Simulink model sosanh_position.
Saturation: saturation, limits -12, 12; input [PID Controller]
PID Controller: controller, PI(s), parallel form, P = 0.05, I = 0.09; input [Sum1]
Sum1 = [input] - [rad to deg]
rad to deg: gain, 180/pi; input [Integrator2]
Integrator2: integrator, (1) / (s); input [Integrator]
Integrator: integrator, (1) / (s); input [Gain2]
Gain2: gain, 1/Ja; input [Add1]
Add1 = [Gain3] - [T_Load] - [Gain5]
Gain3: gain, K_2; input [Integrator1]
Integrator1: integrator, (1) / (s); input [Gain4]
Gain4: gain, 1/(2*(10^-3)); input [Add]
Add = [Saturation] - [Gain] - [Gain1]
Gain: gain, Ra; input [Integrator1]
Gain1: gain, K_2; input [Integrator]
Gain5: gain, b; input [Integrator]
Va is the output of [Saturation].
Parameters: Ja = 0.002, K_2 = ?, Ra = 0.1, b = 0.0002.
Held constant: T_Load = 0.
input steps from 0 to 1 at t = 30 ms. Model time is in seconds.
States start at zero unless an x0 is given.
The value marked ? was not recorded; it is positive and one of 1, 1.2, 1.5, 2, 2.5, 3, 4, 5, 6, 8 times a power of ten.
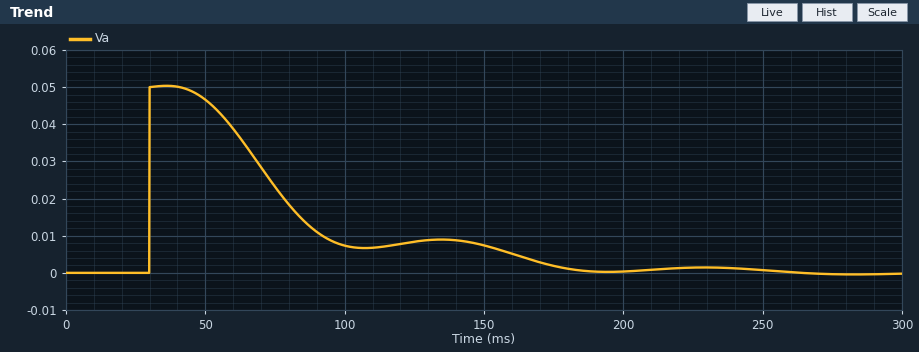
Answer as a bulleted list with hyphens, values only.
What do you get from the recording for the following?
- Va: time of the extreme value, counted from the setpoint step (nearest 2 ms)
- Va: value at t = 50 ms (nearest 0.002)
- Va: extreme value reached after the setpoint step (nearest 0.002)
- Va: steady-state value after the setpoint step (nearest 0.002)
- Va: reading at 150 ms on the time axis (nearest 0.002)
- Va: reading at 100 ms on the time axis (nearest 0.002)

- 6 ms
- 0.046
- 0.050
- 0.000
- 0.008
- 0.008
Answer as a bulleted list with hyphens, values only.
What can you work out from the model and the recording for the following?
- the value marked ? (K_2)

- 0.15
